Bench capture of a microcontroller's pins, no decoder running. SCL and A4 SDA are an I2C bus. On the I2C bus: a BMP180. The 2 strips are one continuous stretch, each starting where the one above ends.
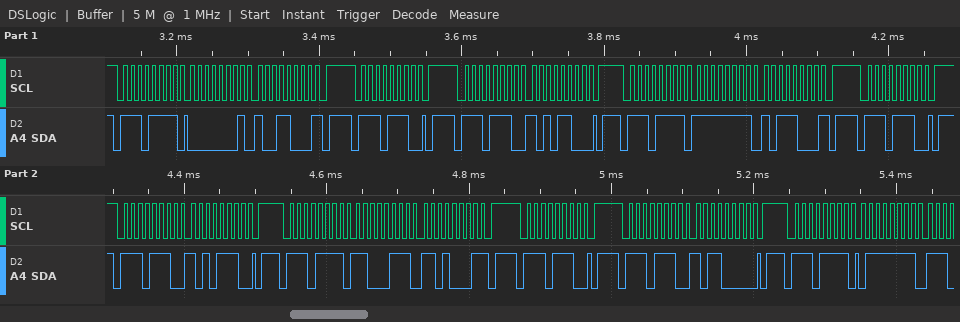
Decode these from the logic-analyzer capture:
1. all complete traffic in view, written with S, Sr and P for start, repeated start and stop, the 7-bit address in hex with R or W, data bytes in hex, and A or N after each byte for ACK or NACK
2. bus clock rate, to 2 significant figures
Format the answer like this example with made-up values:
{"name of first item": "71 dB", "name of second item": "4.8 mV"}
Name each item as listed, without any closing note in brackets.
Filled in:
{"all complete traffic in view, written with S, Sr and P for start, repeated start and stop, the 7-bit address in hex with R or W, data bytes in hex, and A or N after each byte for ACK or NACK": "S 77R A 01 A 98 N P S 77W A P S 77W A AC A P S 77R A FF A B8 N P S 77W A P S 77W A AE A P S 77R A C7 A D1 N P S 77W A P S 77W A B0 A P S 77R A 7F A", "bus clock rate, to 2 significant figures": "100 kHz"}
